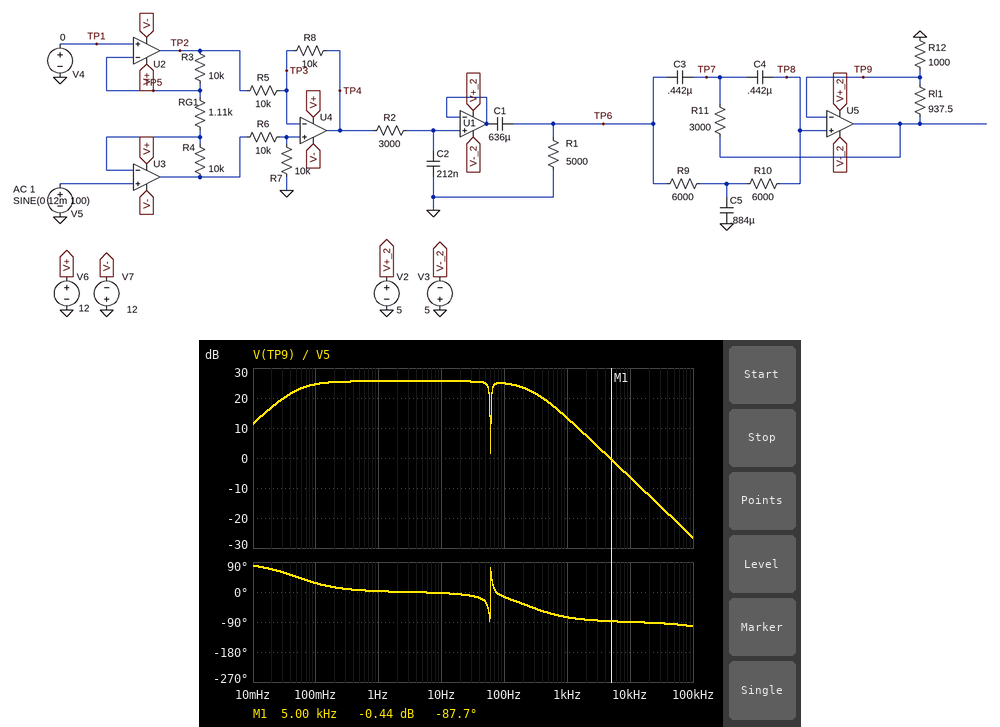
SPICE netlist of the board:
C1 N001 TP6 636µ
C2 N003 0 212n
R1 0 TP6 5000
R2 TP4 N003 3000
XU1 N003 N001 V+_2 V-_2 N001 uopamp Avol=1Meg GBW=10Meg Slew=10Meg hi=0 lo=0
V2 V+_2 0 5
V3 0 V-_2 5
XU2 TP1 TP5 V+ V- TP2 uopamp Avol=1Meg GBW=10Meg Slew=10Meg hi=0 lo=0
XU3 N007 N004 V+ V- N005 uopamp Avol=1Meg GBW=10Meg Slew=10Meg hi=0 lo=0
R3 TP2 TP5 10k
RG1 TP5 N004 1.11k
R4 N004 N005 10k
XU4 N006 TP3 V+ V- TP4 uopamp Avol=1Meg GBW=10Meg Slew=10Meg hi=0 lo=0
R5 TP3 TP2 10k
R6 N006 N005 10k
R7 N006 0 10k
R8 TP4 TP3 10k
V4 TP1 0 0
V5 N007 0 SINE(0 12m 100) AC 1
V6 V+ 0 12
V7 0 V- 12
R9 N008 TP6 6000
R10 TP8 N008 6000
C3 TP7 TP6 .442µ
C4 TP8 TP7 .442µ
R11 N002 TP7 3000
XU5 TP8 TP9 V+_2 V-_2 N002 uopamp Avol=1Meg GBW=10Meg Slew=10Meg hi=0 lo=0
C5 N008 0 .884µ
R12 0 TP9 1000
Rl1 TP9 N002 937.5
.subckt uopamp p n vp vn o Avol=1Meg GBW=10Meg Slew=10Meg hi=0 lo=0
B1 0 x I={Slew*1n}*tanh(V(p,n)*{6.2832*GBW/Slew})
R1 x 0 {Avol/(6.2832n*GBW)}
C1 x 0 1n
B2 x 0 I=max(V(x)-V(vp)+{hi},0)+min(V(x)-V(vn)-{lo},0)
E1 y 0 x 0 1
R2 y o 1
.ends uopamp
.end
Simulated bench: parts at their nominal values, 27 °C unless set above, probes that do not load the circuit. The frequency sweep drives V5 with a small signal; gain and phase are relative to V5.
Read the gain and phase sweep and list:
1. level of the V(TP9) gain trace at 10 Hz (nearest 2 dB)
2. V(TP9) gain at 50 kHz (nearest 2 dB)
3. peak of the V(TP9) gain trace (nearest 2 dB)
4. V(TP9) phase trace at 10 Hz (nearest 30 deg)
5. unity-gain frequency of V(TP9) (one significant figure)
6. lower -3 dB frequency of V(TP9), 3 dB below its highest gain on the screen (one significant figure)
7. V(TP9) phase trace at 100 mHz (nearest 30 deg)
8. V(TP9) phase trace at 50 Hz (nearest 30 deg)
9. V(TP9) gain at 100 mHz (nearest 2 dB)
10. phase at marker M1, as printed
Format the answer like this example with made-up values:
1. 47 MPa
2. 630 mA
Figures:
1. 26 dB
2. -20 dB
3. 26 dB
4. 0 deg
5. 5 kHz
6. 50 mHz
7. 30 deg
8. -30 deg
9. 24 dB
10. -87.7 deg
